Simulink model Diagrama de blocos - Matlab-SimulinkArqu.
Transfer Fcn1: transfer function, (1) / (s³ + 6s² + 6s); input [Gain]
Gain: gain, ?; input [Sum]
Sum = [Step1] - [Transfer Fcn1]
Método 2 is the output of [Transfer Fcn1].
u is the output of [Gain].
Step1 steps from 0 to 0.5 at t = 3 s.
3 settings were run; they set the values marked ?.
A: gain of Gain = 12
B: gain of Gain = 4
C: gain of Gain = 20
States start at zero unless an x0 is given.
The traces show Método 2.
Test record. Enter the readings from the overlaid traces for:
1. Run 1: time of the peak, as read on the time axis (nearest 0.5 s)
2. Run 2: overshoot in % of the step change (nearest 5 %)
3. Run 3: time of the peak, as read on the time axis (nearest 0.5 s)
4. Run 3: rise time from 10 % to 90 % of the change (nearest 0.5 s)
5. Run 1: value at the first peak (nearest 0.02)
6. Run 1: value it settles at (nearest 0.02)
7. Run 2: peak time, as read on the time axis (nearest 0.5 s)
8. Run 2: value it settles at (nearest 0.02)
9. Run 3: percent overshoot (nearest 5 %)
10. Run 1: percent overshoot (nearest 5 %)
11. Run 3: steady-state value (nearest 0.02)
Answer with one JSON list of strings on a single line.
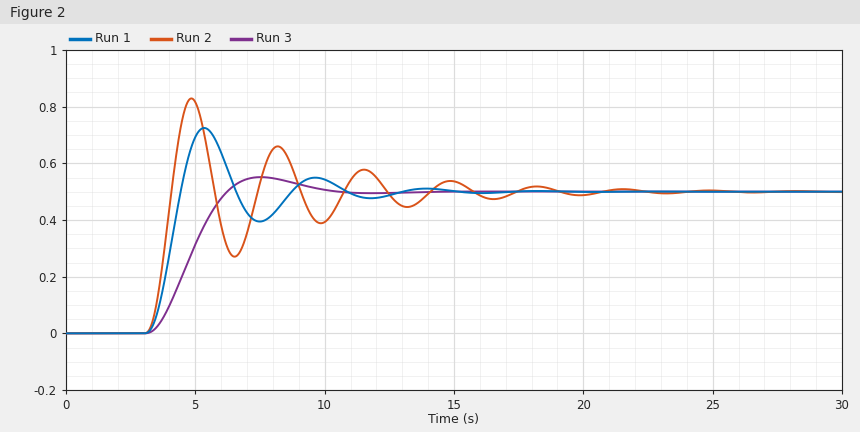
["5.5 s", "65 %", "7.5 s", "2.0 s", "0.72", "0.50", "5.0 s", "0.50", "10 %", "45 %", "0.50"]
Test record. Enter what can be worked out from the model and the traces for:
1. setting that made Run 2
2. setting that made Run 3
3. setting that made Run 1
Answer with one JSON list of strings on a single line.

["C", "B", "A"]
